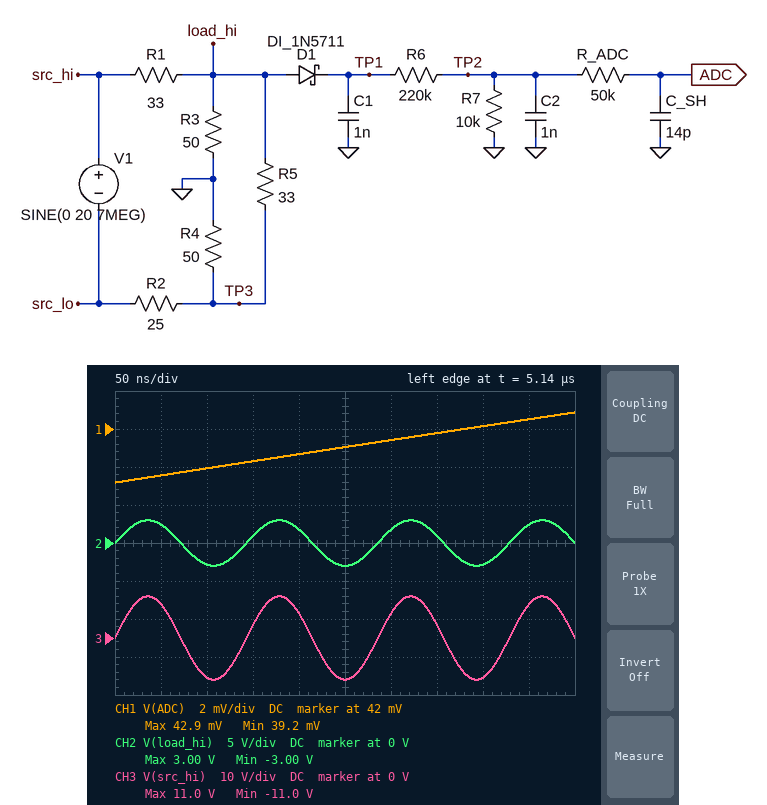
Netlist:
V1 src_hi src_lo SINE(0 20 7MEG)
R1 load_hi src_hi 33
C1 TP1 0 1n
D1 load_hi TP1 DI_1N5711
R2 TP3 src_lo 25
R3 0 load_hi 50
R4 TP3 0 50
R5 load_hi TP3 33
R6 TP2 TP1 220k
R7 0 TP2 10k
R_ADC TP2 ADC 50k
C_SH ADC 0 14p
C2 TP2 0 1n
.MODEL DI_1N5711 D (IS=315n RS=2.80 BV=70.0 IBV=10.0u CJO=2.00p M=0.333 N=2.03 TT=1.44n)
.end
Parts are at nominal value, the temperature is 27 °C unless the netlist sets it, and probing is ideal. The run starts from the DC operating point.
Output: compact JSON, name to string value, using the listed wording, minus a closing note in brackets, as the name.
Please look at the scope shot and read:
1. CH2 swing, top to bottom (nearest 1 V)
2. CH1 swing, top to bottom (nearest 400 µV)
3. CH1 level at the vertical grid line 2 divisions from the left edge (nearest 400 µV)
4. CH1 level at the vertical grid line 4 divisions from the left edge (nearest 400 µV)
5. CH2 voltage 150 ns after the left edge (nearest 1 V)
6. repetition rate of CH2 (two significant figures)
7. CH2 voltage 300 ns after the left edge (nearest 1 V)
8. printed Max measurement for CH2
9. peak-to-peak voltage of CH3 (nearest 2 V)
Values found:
{"CH2 swing, top to bottom": "6 V", "CH1 swing, top to bottom": "3.6 mV", "CH1 level at the vertical grid line 2 divisions from the left edge": "40.0 mV", "CH1 level at the vertical grid line 4 divisions from the left edge": "40.8 mV", "CH2 voltage 150 ns after the left edge": "1 V", "repetition rate of CH2": "7.0 MHz", "CH2 voltage 300 ns after the left edge": "2 V", "printed Max measurement for CH2": "3.00 V", "peak-to-peak voltage of CH3": "22 V"}
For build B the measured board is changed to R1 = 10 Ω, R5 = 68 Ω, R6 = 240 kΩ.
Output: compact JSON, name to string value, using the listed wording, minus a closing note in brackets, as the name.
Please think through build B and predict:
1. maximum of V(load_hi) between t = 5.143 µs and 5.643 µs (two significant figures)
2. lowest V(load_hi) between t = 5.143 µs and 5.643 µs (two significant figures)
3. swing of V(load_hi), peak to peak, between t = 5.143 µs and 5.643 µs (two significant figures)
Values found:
{"maximum of V(load_hi) between t = 5.143 µs and 5.643 µs": "5.3 V", "lowest V(load_hi) between t = 5.143 µs and 5.643 µs": "-5.4 V", "swing of V(load_hi), peak to peak, between t = 5.143 µs and 5.643 µs": "11 V"}
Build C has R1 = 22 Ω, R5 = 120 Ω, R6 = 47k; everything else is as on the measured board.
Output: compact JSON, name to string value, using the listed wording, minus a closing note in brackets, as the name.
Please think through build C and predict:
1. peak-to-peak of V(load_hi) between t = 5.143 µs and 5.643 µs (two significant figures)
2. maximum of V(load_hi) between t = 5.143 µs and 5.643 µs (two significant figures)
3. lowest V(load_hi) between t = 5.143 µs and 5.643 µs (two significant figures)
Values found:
{"peak-to-peak of V(load_hi) between t = 5.143 µs and 5.643 µs": "11 V", "maximum of V(load_hi) between t = 5.143 µs and 5.643 µs": "5.3 V", "lowest V(load_hi) between t = 5.143 µs and 5.643 µs": "-5.4 V"}
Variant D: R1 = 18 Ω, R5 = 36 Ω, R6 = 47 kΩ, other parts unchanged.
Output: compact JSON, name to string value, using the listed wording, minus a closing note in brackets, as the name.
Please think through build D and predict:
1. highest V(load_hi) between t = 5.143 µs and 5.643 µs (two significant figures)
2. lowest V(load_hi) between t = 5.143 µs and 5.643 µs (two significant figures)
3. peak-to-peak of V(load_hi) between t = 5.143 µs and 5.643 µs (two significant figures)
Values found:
{"highest V(load_hi) between t = 5.143 µs and 5.643 µs": "3.8 V", "lowest V(load_hi) between t = 5.143 µs and 5.643 µs": "-3.8 V", "peak-to-peak of V(load_hi) between t = 5.143 µs and 5.643 µs": "7.6 V"}
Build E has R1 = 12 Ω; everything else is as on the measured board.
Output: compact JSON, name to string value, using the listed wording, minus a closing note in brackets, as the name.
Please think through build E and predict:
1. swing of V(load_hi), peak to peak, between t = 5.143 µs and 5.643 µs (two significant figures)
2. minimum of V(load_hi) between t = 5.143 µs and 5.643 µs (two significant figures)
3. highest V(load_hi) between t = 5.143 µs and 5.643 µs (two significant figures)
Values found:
{"swing of V(load_hi), peak to peak, between t = 5.143 µs and 5.643 µs": "8.0 V", "minimum of V(load_hi) between t = 5.143 µs and 5.643 µs": "-4.0 V", "highest V(load_hi) between t = 5.143 µs and 5.643 µs": "4.0 V"}
